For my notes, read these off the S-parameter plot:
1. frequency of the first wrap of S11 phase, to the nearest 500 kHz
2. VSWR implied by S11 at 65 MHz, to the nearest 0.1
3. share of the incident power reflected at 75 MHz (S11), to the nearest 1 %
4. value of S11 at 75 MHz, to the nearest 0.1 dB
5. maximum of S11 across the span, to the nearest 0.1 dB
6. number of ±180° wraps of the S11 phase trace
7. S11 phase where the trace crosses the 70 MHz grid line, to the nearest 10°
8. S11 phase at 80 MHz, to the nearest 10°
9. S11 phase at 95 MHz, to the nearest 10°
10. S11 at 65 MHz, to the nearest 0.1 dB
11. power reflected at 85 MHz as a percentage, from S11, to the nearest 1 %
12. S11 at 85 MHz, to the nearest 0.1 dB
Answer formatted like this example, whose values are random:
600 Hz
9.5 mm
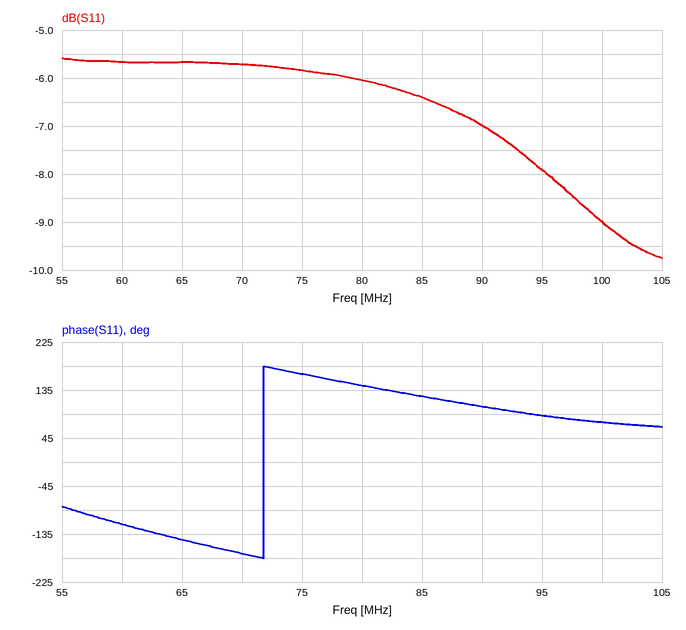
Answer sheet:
72.0 MHz
3.2
26 %
-5.8 dB
-5.6 dB
1
-170°
140°
90°
-5.7 dB
23 %
-6.4 dB
